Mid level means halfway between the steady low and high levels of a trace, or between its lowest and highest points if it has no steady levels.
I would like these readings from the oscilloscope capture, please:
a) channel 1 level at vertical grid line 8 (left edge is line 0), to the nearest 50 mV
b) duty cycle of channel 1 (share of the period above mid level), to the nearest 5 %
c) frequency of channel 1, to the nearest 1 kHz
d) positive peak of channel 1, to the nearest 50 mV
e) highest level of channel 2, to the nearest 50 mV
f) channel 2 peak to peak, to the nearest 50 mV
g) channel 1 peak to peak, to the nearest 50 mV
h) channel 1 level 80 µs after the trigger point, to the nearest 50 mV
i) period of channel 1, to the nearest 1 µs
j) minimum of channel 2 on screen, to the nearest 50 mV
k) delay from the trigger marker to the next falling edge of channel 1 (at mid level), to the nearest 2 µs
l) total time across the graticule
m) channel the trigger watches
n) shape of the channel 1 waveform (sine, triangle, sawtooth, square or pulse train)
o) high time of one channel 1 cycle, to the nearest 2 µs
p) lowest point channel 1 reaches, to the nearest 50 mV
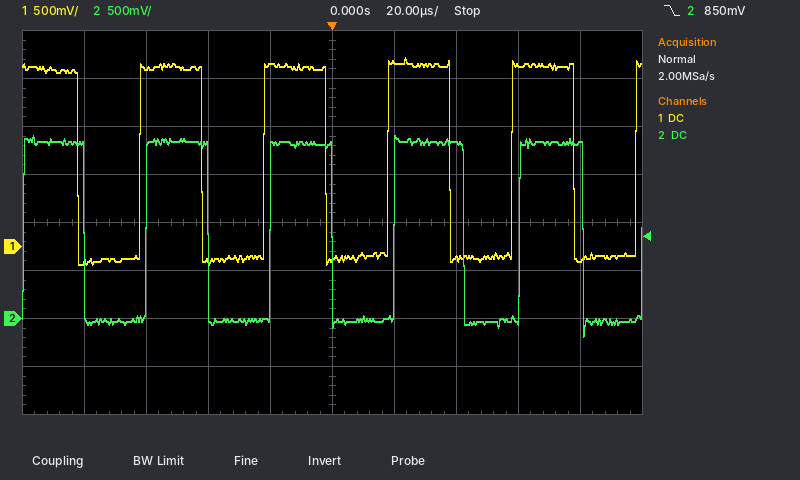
1.90 V
50 %
25 kHz
1.95 V
1.90 V
2.10 V
2.15 V
-150 mV
40 µs
-200 mV
38 µs
200 µs
channel 2
square
20 µs
-200 mV
